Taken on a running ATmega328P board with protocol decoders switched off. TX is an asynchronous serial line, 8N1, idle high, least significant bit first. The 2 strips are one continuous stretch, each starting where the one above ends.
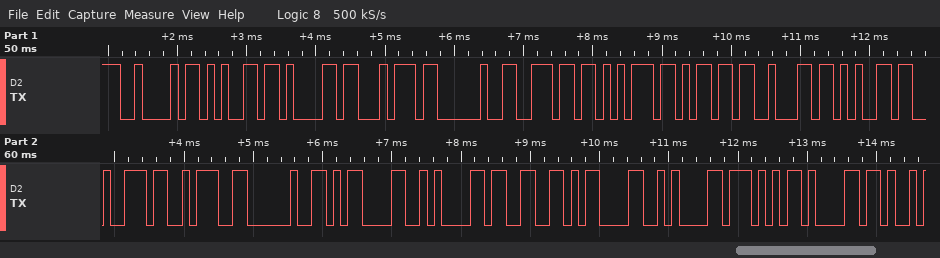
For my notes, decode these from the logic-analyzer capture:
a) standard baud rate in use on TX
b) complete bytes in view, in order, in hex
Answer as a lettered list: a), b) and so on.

a) 9600 baud
b) 42 65 61 74 20 6E 75 6D 62 65 72 3A 20 0D 0A 33 0D 0A 57 61
